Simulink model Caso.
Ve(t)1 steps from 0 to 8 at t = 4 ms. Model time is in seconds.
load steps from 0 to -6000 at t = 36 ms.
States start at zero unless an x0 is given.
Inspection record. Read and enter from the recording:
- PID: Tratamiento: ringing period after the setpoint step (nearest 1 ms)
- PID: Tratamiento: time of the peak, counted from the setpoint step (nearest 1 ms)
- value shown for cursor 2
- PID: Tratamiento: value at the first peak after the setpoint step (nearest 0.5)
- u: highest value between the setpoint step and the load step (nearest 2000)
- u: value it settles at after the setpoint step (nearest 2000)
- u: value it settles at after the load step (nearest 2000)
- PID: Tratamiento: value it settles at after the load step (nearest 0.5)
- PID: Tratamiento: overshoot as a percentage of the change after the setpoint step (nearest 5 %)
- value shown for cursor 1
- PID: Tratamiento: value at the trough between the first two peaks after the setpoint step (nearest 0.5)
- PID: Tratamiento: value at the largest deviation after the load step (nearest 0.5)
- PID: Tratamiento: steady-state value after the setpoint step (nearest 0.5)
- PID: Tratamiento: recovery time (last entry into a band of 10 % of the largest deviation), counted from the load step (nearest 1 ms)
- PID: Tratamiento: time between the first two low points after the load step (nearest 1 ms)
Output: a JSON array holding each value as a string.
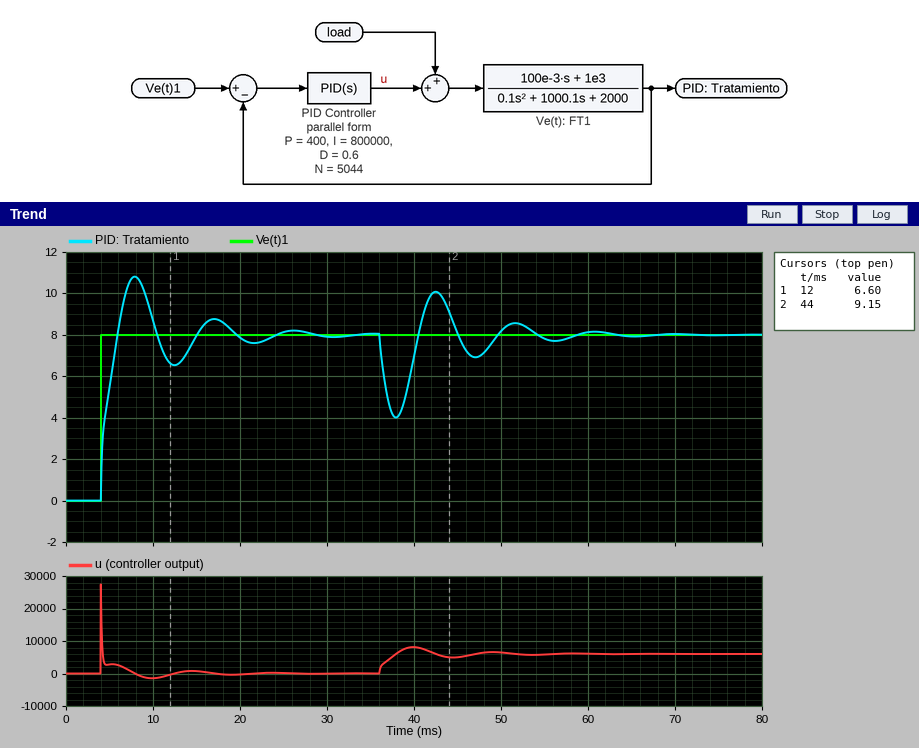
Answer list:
["9 ms", "4 ms", "9.15", "11.0", "28000", "0", "6000", "8.0", "35 %", "6.60", "6.5", "4.0", "8.0", "17 ms", "9 ms"]
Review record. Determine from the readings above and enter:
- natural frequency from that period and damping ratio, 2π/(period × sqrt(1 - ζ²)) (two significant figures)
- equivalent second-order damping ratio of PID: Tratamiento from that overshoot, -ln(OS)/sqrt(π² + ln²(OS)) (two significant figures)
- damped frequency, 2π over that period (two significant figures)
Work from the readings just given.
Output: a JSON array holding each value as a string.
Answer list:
["0.74 rad/ms", "0.32", "0.70 rad/ms"]
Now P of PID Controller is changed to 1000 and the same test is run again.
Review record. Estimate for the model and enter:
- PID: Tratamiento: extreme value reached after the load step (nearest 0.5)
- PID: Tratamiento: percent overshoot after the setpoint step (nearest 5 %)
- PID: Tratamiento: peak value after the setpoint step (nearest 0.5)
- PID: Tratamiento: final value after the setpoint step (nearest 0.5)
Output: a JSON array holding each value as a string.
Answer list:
["5.0", "20 %", "9.5", "8.0"]
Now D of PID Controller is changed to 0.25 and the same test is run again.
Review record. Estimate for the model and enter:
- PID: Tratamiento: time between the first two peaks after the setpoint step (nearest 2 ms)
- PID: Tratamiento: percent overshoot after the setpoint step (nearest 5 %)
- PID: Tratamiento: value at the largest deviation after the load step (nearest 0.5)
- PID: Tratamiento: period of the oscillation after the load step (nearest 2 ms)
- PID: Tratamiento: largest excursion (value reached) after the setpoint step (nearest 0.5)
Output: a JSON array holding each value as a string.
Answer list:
["8 ms", "45 %", "3.5", "8 ms", "11.5"]
